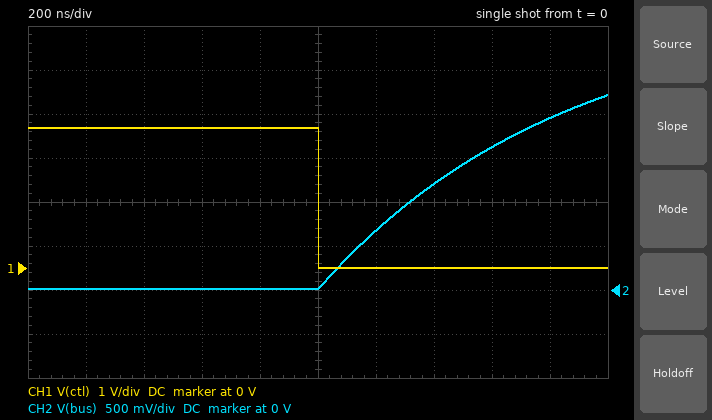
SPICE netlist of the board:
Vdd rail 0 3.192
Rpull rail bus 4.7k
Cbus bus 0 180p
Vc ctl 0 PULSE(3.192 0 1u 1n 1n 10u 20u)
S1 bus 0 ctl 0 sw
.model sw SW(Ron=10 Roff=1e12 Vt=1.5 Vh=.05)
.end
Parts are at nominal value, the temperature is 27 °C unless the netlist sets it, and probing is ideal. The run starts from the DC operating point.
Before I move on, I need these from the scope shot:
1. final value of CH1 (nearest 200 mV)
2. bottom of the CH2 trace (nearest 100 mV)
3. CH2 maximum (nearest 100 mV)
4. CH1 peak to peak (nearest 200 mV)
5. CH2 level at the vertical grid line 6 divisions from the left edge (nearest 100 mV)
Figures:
0 V
0 V
2.2 V
3.2 V
700 mV
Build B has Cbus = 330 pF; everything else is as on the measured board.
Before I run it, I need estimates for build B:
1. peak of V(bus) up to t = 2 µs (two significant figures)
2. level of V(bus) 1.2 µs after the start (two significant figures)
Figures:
1.5 V
390 mV
